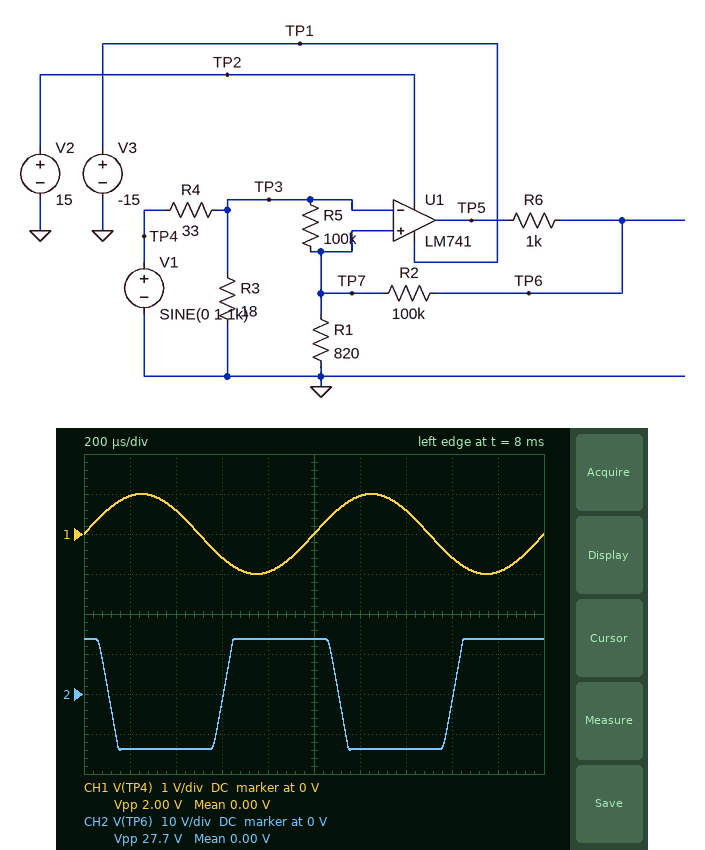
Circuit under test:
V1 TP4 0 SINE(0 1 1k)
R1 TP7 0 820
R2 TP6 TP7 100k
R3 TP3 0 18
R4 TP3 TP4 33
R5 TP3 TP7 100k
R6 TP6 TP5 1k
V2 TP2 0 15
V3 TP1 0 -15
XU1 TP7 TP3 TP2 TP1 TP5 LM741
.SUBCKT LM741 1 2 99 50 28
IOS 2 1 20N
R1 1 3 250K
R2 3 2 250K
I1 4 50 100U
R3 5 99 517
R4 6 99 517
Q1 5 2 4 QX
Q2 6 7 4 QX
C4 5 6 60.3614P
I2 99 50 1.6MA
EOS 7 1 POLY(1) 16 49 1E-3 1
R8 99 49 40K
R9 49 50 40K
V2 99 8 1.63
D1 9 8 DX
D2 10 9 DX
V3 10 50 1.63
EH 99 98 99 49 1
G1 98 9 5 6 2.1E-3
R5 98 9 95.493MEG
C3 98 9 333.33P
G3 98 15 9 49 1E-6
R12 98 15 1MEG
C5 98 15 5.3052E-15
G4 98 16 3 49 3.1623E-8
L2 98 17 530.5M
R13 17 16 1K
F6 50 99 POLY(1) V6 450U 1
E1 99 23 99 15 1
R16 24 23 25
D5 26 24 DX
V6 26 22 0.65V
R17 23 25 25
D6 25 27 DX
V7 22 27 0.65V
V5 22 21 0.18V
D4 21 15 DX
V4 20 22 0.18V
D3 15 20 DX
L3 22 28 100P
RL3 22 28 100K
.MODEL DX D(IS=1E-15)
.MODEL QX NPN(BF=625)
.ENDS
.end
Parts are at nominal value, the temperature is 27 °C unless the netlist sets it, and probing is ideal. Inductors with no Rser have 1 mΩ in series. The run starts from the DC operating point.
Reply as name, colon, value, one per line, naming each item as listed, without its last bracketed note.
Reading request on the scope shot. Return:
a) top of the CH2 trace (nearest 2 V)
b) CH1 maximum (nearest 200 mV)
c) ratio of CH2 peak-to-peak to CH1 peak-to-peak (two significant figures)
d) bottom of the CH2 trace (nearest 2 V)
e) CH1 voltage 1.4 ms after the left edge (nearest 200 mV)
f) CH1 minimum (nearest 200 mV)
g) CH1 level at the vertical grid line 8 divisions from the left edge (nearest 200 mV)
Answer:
top of the CH2 trace: 14 V
CH1 maximum: 1.0 V
ratio of CH2 peak-to-peak to CH1 peak-to-peak: 14
bottom of the CH2 trace: -14 V
CH1 voltage 1.4 ms after the left edge: 600 mV
CH1 minimum: -1.0 V
CH1 level at the vertical grid line 8 divisions from the left edge: -600 mV
